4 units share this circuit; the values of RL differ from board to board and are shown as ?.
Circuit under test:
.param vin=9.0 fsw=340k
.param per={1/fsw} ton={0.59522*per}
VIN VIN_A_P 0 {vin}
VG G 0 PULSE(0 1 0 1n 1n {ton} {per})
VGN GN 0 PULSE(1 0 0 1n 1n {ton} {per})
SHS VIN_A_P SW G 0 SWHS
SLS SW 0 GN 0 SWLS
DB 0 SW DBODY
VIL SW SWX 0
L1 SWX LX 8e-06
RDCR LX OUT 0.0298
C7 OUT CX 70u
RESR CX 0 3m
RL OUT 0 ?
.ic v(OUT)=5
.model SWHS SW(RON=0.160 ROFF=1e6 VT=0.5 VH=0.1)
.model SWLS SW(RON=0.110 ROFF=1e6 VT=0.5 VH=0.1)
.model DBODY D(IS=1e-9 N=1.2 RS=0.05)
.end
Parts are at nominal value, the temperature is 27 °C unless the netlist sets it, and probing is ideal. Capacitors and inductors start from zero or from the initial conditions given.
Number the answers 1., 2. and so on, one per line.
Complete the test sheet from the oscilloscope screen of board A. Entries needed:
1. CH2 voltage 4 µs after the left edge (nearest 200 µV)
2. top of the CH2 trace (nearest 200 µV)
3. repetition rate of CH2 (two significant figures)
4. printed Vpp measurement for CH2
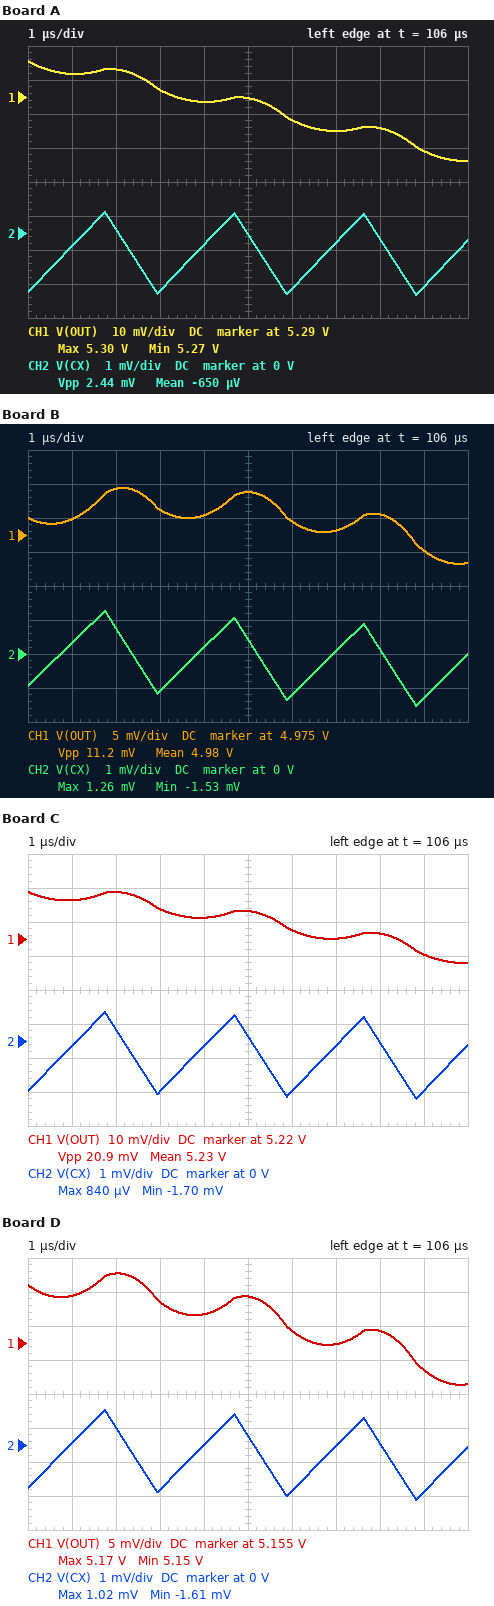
1. -400 µV
2. 600 µV
3. 340 kHz
4. 2.44 mV
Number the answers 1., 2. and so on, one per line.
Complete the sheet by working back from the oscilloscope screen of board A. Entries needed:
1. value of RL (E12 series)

1. 6.8 Ω
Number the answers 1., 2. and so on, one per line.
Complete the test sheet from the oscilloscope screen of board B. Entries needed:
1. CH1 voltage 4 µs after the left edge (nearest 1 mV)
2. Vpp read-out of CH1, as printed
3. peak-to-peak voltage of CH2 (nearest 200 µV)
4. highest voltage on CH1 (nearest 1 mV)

1. 4.978 V
2. 11.2 mV
3. 2.8 mV
4. 4.982 V
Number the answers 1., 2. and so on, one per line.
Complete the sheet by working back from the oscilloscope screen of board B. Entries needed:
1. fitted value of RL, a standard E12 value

1. 1.5 Ω
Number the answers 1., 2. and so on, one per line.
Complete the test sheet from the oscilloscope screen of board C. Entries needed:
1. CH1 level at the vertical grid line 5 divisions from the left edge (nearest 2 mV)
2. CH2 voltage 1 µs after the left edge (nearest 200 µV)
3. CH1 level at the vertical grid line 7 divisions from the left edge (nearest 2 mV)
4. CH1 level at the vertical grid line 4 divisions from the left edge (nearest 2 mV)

1. 5.228 V
2. -200 µV
3. 5.220 V
4. 5.226 V
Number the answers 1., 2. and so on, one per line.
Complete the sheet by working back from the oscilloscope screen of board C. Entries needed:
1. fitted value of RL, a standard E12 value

1. 3.9 Ω
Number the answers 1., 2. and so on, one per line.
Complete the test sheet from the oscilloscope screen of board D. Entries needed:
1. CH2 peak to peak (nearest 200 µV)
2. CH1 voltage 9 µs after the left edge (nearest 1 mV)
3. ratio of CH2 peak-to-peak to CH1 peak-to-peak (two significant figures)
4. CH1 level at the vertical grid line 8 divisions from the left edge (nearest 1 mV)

1. 2.6 mV
2. 5.151 V
3. 0.16
4. 5.157 V
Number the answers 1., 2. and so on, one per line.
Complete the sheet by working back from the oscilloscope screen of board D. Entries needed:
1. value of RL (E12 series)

1. 2.7 Ω
